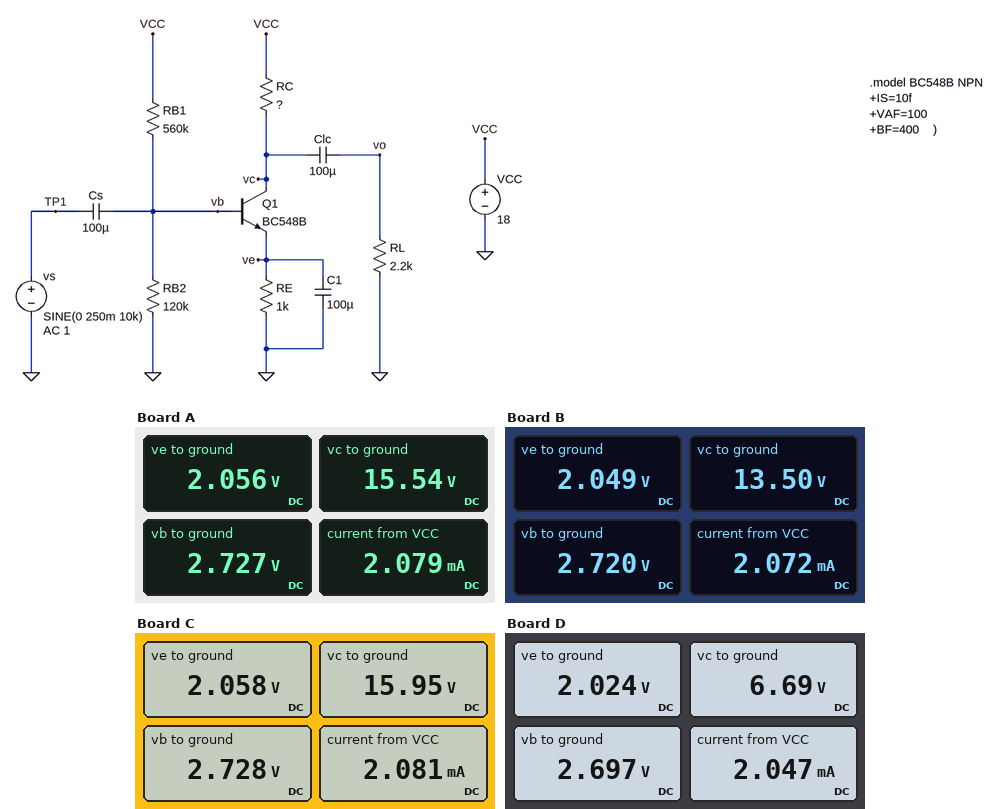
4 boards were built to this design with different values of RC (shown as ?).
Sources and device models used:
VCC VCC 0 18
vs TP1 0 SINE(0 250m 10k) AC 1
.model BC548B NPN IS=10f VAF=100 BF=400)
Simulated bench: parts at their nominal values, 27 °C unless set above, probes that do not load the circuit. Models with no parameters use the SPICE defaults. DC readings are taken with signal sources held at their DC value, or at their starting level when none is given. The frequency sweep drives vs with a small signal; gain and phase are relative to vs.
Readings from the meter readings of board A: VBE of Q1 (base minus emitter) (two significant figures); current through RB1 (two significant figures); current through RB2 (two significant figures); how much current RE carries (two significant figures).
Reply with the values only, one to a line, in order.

670 mV
27 µA
23 µA
2.1 mA
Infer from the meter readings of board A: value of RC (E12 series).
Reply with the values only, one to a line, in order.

1.2 kΩ
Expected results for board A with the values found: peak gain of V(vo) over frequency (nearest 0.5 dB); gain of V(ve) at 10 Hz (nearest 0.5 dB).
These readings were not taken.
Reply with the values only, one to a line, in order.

35.5 dB
0 dB
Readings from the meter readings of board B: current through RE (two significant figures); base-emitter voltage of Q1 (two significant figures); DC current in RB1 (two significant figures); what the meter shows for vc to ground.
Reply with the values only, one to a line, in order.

2.0 mA
670 mV
27 µA
13.50 V
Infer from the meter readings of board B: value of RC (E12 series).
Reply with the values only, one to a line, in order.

2.2 kΩ
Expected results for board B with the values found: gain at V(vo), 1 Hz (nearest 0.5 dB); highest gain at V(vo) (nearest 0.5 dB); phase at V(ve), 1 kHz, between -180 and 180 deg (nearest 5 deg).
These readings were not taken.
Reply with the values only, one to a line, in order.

1.5 dB
38.5 dB
-85 deg
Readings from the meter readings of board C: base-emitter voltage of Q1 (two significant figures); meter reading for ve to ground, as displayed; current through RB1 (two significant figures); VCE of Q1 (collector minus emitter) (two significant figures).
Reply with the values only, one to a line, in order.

670 mV
2.058 V
27 µA
14 V
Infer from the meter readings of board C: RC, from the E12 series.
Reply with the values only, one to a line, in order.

1 kΩ
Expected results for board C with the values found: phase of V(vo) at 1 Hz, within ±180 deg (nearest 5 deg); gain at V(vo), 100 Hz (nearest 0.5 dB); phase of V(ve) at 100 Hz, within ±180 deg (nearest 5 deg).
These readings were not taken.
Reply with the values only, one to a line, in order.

-120 deg
30.5 dB
-40 deg
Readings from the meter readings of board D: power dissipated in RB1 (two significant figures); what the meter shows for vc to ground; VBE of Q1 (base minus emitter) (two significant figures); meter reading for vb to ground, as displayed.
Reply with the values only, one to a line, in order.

420 µW
6.69 V
670 mV
2.697 V
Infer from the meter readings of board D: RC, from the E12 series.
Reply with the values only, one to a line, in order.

5.6 kΩ
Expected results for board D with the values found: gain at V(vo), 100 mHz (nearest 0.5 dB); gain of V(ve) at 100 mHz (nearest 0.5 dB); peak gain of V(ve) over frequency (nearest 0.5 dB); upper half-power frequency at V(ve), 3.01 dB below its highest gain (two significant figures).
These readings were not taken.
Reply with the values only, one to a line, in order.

-3.5 dB
-0.5 dB
0 dB
120 Hz
